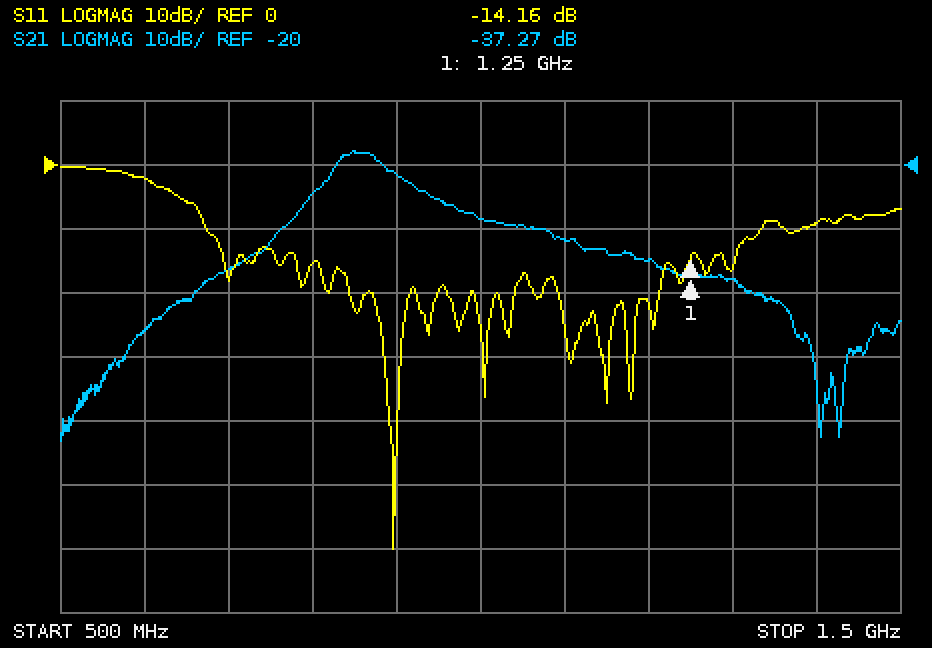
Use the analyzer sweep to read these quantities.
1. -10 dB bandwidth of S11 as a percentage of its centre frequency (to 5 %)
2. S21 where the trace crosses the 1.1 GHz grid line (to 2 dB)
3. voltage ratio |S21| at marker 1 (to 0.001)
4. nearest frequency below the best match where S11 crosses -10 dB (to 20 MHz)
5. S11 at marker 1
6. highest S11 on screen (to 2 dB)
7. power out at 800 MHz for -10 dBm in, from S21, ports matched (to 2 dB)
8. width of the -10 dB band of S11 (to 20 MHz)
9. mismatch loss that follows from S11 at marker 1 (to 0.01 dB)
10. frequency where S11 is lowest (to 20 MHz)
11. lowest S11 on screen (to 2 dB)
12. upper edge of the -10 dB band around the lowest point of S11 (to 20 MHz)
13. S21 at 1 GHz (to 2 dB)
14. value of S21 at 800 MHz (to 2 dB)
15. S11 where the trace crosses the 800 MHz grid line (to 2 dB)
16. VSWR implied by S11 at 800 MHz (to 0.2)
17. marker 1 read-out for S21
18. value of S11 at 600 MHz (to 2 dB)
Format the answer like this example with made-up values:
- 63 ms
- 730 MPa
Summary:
- 65 %
- -32 dB
- 0.014
- 680 MHz
- -14.16 dB
- 0 dB
- -34 dBm
- 660 MHz
- 0.17 dB
- 900 MHz
- -60 dB
- 1.34 GHz
- -28 dB
- -24 dB
- -16 dB
- 1.4
- -37.27 dB
- -2 dB
